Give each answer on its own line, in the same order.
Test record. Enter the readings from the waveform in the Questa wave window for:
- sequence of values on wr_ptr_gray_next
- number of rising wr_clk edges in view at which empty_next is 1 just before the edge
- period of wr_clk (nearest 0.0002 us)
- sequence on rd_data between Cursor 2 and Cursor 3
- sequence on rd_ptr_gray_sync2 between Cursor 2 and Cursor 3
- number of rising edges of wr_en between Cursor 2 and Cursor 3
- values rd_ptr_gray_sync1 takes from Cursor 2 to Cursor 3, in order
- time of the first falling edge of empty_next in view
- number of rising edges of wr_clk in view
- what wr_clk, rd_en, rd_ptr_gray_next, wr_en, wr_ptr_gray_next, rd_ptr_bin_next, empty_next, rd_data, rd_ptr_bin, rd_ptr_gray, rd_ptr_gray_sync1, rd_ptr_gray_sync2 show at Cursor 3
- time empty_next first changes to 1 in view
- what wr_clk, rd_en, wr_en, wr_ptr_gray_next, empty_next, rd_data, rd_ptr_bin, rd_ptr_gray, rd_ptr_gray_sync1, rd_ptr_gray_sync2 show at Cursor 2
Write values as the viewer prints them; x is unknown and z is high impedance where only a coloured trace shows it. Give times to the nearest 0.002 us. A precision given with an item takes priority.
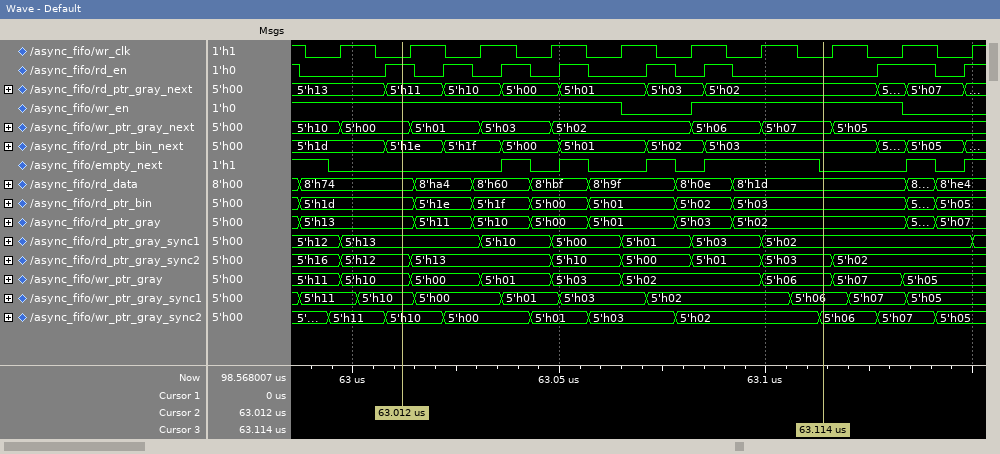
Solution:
5'h10, 5'h00, 5'h01, 5'h03, 5'h02, 5'h06, 5'h07, 5'h05
2
0.017 us
8'h74, 8'ha4, 8'h60, 8'hbf, 8'h9f, 8'h0e, 8'h1d
5'h12, 5'h13, 5'h10, 5'h00, 5'h01, 5'h03
1
5'h13, 5'h10, 5'h00, 5'h01, 5'h03, 5'h02
62.994 us
10
wr_clk=0, rd_en=0, rd_ptr_gray_next=5'h02, wr_en=1, wr_ptr_gray_next=5'h07, rd_ptr_bin_next=5'h03, empty_next=0, rd_data=8'h1d, rd_ptr_bin=5'h03, rd_ptr_gray=5'h02, rd_ptr_gray_sync1=5'h02, rd_ptr_gray_sync2=5'h03
63.036 us
wr_clk=0, rd_en=1, wr_en=1, wr_ptr_gray_next=5'h00, empty_next=0, rd_data=8'h74, rd_ptr_bin=5'h1d, rd_ptr_gray=5'h13, rd_ptr_gray_sync1=5'h13, rd_ptr_gray_sync2=5'h12
